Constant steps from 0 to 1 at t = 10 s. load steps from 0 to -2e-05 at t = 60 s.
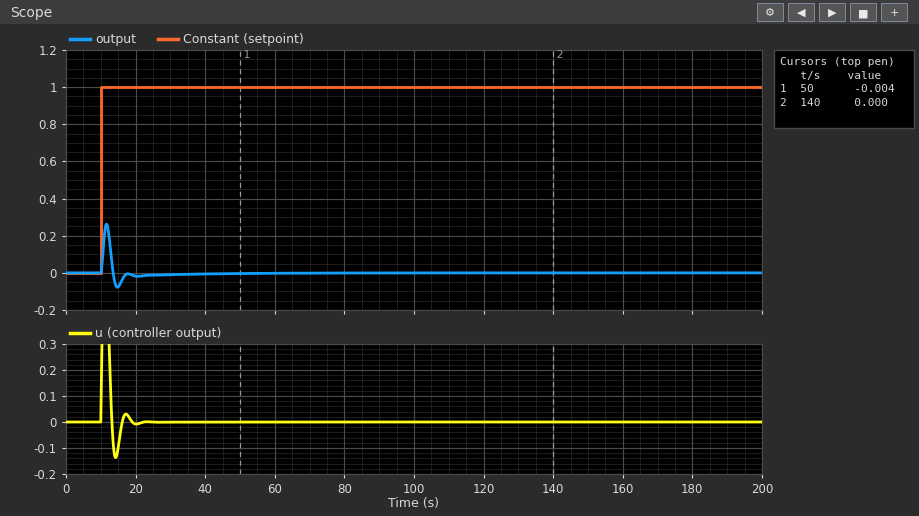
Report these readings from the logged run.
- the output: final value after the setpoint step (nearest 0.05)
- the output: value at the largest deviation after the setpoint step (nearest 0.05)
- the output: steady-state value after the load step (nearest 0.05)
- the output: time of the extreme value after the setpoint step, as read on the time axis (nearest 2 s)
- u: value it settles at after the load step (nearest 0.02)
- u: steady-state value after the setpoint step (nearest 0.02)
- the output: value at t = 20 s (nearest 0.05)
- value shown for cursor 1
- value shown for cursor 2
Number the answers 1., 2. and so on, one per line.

1. 0.00
2. 0.25
3. 0.00
4. 12 s
5. 0.00
6. 0.00
7. 0.00
8. -0.004
9. 0.000
